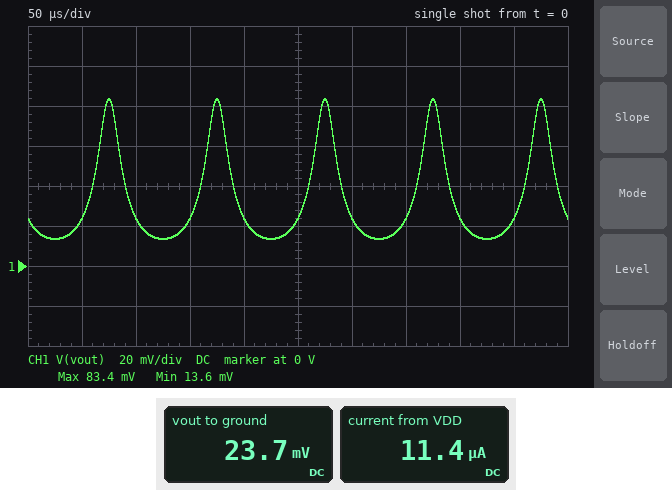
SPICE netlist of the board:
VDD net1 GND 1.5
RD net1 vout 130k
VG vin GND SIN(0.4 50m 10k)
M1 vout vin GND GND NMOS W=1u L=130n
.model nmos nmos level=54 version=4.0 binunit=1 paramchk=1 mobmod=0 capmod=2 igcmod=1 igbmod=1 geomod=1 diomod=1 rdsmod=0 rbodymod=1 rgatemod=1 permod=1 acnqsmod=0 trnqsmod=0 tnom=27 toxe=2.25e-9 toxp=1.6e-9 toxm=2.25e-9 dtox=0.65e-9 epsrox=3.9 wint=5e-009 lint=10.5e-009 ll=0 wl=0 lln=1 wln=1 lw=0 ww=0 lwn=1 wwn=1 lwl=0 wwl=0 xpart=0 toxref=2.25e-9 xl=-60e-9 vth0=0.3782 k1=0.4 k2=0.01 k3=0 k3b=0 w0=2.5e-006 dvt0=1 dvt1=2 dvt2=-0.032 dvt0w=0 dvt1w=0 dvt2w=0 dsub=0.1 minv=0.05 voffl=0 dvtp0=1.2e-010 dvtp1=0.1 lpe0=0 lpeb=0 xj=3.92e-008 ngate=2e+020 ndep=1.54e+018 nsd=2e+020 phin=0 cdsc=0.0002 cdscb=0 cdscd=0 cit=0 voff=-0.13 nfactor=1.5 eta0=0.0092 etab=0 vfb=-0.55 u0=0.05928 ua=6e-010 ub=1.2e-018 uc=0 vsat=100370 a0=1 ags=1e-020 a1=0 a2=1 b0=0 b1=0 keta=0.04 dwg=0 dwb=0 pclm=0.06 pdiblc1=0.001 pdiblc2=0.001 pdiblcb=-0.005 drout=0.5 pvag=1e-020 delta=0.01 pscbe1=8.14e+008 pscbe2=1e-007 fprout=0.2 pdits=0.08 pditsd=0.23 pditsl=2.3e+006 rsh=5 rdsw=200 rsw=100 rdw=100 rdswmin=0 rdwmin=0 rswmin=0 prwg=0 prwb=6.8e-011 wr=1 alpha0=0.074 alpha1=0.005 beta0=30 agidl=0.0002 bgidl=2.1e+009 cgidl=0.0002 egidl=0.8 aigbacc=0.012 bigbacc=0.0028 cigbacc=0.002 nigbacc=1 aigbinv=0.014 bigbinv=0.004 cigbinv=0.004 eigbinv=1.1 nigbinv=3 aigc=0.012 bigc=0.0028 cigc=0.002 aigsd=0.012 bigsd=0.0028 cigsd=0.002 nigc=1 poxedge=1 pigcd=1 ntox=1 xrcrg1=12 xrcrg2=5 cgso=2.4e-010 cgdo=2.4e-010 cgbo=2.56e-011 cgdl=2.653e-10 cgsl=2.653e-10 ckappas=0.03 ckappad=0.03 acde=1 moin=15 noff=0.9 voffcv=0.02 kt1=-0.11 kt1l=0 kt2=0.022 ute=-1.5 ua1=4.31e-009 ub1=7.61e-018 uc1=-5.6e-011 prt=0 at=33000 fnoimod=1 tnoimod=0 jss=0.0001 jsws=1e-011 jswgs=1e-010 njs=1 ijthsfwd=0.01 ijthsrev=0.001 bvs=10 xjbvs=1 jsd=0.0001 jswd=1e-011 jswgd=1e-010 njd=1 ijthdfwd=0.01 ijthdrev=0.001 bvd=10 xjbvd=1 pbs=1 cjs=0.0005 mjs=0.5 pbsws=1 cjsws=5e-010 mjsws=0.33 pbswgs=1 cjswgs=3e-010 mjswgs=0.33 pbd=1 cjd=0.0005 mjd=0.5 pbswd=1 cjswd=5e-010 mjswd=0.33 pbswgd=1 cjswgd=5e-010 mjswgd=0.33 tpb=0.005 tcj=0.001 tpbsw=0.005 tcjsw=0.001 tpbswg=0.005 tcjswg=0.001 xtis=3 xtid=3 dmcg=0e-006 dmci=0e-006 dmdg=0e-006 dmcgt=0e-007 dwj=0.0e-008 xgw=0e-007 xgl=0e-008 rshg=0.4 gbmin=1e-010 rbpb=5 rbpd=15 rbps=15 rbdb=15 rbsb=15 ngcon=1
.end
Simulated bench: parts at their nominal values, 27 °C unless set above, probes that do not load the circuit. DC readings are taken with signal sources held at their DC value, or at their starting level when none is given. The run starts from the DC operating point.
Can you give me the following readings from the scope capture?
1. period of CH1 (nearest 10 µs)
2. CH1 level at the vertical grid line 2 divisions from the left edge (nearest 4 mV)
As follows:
100 µs
24 mV
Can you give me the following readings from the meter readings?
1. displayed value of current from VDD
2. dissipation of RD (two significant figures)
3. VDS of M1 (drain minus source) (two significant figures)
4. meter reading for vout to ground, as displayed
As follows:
11.4 µA
17 µW
24 mV
23.7 mV
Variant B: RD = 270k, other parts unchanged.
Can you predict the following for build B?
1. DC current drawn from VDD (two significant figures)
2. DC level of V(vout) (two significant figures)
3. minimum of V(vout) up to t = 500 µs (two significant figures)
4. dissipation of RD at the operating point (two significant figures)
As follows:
5.5 µA
10 mV
6.3 mV
8.2 µW
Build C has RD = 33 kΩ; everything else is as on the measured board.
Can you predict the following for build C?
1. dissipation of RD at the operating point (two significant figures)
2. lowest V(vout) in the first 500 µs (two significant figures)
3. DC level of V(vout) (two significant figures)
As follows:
42 µW
79 mV
330 mV
